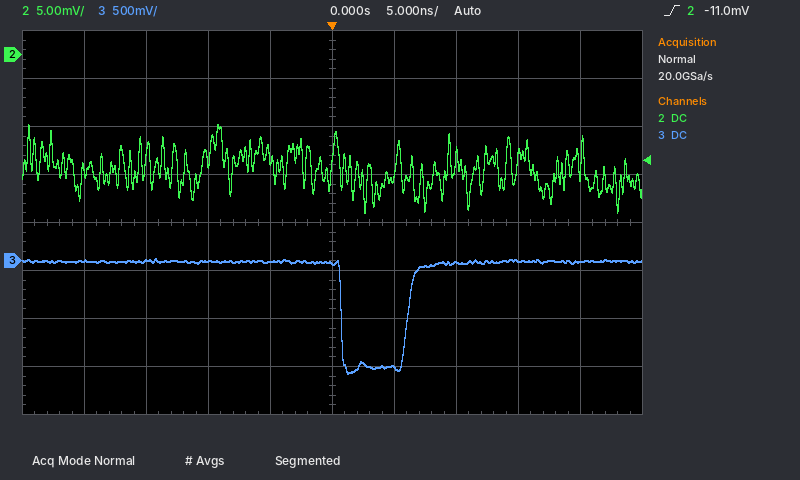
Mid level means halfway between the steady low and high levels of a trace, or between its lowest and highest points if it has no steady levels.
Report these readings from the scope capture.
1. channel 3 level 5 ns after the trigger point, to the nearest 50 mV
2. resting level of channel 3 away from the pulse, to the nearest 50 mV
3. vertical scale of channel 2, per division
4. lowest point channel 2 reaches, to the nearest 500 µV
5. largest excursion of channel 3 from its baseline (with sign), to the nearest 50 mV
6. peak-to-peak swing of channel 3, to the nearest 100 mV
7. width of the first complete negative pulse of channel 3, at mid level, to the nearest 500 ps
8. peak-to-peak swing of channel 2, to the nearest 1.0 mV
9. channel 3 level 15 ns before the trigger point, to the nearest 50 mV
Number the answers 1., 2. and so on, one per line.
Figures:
1. -1.10 V
2. 0 mV
3. 5 mV
4. -16.5 mV
5. -1.15 V
6. 1.20 V
7. 5.5 ns
8. 9.0 mV
9. 0 mV
